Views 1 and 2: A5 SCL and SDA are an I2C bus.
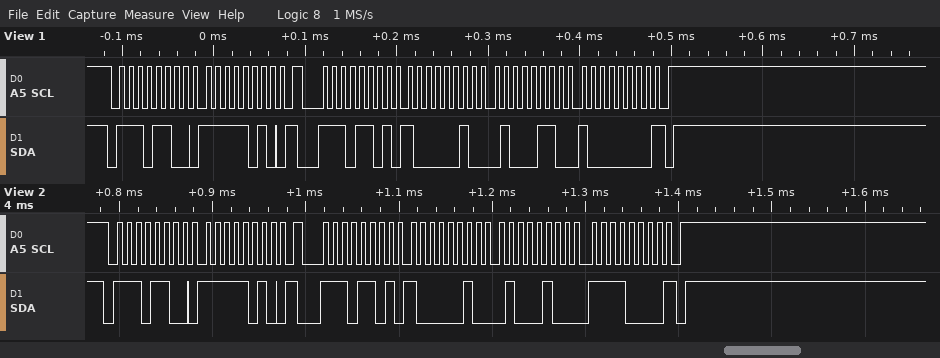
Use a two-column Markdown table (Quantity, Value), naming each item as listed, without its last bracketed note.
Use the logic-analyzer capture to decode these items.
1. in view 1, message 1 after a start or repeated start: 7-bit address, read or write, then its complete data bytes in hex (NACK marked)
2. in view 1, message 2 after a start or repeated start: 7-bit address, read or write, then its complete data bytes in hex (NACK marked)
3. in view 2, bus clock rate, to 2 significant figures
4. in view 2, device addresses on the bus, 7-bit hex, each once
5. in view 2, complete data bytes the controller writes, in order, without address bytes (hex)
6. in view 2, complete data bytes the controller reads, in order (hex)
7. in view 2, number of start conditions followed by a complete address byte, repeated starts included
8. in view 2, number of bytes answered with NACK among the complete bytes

| Quantity | Value |
|---|---|
| in view 1, message 1 after a start or repeated start: 7-bit address, read or write, then its complete data bytes in hex | 0x76 write: FA |
| in view 1, message 2 after a start or repeated start: 7-bit address, read or write, then its complete data bytes in hex | 0x76 read: 82 46 80 NACK |
| in view 2, bus clock rate, to 2 significant figures | 100 kHz |
| in view 2, device addresses on the bus, 7-bit hex, each once | 0x76 |
| in view 2, complete data bytes the controller writes, in order, without address bytes | FA |
| in view 2, complete data bytes the controller reads, in order | 82 44 F0 |
| in view 2, number of start conditions followed by a complete address byte, repeated starts included | 2 |
| in view 2, number of bytes answered with NACK among the complete bytes | 1 |
